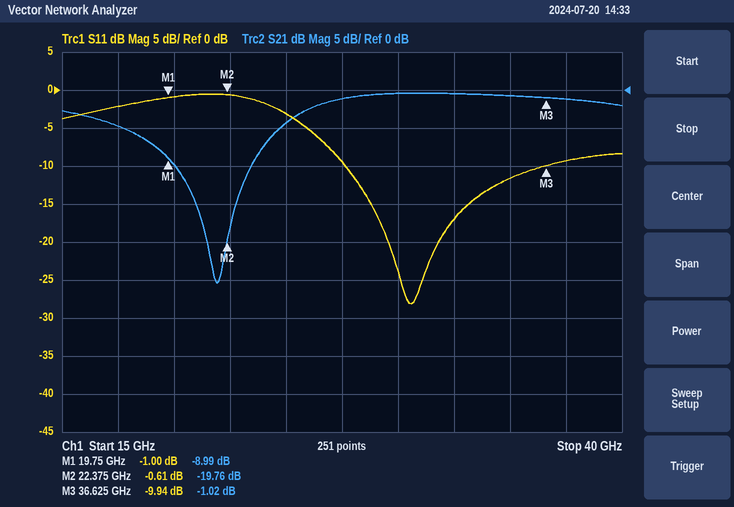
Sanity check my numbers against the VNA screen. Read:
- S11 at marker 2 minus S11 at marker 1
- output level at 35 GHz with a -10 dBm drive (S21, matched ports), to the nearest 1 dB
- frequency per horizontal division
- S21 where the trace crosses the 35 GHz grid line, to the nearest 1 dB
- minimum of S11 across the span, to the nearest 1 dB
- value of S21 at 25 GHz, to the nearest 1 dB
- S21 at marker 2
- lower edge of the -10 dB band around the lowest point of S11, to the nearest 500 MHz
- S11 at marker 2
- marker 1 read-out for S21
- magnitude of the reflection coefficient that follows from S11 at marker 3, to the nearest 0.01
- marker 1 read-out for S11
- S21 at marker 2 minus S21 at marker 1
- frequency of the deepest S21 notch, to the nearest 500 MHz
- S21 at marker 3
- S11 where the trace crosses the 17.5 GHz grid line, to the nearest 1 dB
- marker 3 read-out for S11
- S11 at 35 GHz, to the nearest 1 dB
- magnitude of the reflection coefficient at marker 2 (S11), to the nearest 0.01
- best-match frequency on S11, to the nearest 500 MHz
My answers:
0.39 dB
-11 dBm
2.5 GHz
-1 dB
-28 dB
-4 dB
-19.76 dB
27.5 GHz
-0.61 dB
-8.99 dB
0.32
-1.00 dB
-10.77 dB
22.0 GHz
-1.02 dB
-2 dB
-9.94 dB
-12 dB
0.93
30.5 GHz
